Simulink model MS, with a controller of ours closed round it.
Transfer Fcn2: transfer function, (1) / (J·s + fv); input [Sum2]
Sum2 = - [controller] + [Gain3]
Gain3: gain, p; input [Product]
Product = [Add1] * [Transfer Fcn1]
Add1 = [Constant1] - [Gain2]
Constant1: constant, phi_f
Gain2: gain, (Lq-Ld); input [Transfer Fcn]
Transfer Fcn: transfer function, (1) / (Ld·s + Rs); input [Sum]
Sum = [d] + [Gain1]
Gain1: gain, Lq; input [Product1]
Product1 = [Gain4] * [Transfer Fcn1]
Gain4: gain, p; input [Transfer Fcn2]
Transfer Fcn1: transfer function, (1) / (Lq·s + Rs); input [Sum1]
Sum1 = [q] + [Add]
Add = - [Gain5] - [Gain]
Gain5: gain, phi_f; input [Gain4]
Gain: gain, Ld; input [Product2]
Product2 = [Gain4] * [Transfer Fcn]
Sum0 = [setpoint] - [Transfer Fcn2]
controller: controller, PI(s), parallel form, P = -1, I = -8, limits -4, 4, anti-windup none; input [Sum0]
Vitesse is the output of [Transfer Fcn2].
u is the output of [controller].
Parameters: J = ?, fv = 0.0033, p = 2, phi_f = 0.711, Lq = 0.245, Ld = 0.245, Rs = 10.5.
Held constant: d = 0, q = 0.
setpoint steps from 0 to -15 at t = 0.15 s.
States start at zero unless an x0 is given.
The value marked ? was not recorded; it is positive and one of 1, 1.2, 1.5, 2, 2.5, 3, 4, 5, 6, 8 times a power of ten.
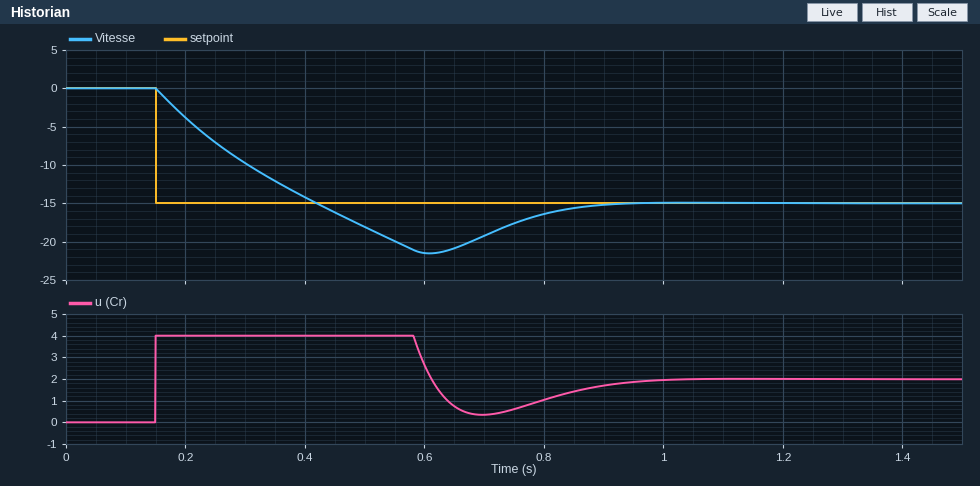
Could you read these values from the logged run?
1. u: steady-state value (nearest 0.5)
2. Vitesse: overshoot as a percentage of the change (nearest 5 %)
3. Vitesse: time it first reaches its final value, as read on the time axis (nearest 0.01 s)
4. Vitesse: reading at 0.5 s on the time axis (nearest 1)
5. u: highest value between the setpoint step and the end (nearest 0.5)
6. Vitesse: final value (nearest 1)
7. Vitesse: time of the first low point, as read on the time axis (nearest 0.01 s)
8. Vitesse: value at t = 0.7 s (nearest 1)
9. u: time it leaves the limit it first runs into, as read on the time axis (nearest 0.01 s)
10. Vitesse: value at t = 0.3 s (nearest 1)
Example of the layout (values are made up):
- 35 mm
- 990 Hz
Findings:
- 2.0
- 45 %
- 0.42 s
- -18
- 4.0
- -15
- 0.61 s
- -19
- 0.58 s
- -10
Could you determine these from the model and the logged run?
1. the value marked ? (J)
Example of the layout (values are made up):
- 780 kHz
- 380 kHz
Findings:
- 0.05
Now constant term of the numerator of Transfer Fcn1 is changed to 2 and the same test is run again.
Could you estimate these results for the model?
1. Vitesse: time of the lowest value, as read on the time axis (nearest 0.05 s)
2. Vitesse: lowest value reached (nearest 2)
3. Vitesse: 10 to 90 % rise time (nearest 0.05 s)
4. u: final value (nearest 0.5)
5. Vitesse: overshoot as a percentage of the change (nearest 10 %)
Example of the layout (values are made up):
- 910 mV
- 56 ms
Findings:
- 0.95 s
- -22
- 0.35 s
- 3.0
- 50 %
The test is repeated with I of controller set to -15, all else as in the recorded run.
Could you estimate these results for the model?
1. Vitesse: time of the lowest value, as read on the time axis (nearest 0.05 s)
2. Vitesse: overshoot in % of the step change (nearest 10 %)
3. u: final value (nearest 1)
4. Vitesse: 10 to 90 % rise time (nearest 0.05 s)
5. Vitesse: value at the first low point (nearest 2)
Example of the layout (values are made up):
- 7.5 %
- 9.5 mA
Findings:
- 0.65 s
- 60 %
- 2
- 0.20 s
- -24
